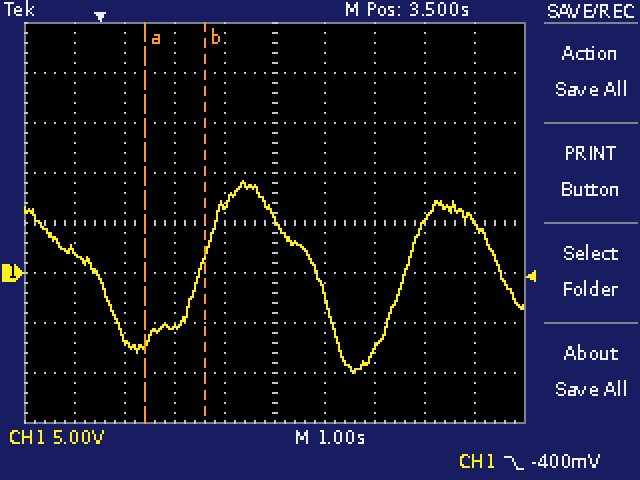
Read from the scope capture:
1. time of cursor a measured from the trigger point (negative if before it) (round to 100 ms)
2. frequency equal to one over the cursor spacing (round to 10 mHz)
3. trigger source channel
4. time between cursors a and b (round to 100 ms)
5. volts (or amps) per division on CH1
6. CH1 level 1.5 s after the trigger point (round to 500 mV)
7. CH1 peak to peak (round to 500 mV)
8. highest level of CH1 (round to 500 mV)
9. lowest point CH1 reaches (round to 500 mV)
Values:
+900 ms
830 mHz
CH1
1.2 s
5 V
-5.5 V
19.0 V
9.0 V
-10.0 V
